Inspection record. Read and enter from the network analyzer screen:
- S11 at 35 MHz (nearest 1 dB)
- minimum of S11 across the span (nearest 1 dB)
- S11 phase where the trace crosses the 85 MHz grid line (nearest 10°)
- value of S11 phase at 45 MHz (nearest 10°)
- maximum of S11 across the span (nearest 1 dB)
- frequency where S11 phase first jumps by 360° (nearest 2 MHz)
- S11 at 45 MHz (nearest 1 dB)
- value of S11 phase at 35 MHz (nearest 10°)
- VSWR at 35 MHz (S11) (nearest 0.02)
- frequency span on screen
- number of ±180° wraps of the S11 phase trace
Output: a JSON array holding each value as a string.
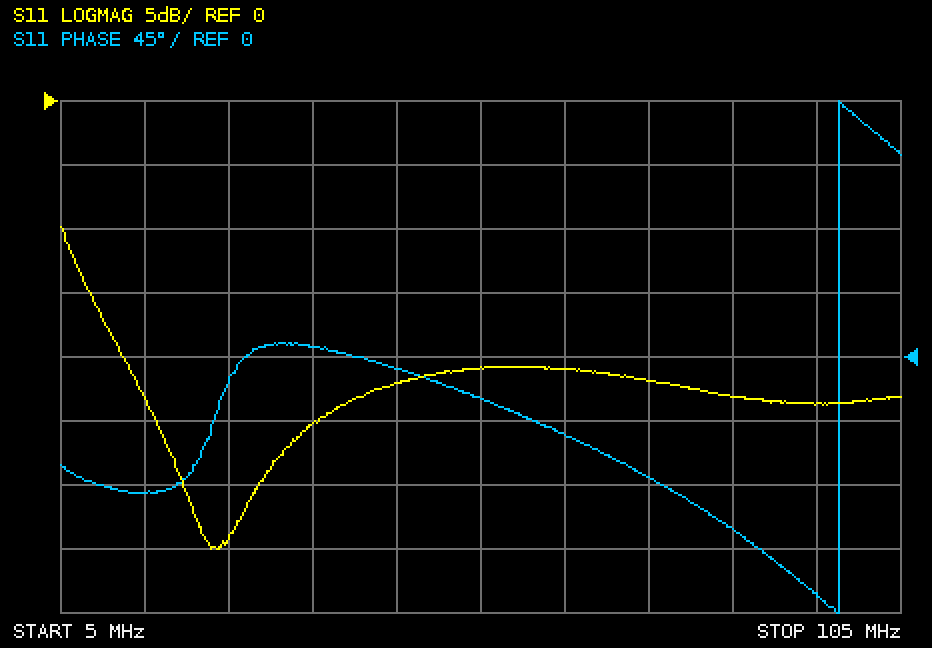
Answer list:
["-25 dB", "-35 dB", "-120°", "-10°", "-10 dB", "98 MHz", "-22 dB", "10°", "1.12", "100 MHz", "1"]
